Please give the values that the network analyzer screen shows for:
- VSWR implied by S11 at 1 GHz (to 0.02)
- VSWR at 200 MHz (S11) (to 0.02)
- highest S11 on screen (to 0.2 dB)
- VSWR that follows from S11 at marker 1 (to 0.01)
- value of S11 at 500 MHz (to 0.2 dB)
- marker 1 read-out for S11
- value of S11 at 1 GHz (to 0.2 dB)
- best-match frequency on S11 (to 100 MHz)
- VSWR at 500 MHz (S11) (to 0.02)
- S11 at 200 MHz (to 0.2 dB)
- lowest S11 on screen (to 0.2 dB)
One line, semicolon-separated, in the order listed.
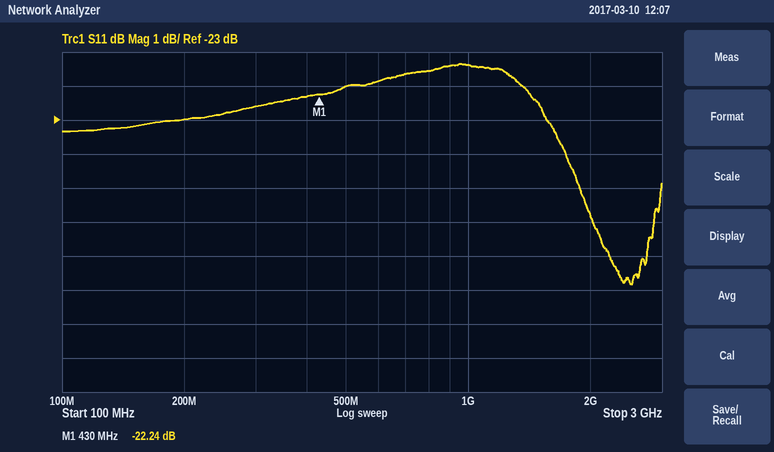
1.18; 1.16; -21.4 dB; 1.17; -22.0 dB; -22.24 dB; -21.4 dB; 2.5 GHz; 1.18; -23.0 dB; -27.8 dB
